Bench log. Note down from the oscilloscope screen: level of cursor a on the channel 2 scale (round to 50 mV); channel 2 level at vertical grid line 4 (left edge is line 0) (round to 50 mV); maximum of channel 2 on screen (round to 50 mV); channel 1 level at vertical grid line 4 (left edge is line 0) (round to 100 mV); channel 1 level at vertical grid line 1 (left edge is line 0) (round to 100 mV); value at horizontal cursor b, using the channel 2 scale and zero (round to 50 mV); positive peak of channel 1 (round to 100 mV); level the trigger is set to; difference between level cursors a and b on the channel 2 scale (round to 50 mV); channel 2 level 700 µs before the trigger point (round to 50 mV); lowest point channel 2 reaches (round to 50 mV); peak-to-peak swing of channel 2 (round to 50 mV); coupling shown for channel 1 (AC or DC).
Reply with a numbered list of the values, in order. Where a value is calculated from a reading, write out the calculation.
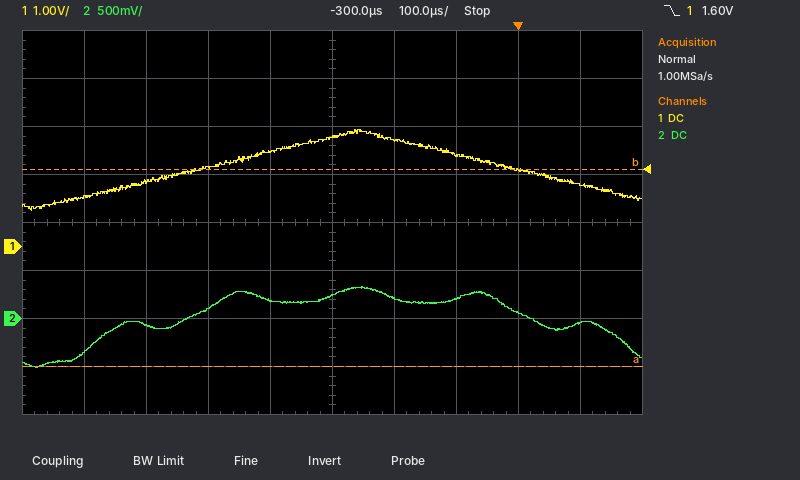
1. -500 mV
2. 200 mV
3. 350 mV
4. 2.0 V
5. 1.0 V
6. 1.55 V
7. 2.4 V
8. 1.60 V
9. 2.05 V
10. -350 mV
11. -500 mV
12. 350 mV − (-500 mV) = 850 mV
13. DC
